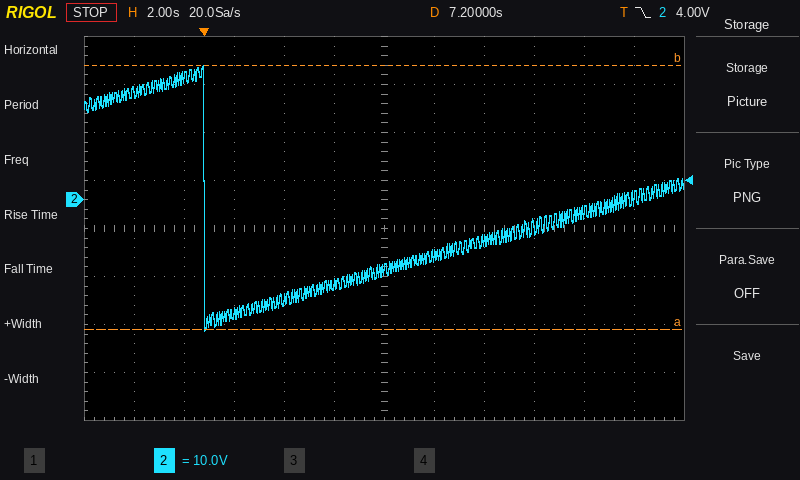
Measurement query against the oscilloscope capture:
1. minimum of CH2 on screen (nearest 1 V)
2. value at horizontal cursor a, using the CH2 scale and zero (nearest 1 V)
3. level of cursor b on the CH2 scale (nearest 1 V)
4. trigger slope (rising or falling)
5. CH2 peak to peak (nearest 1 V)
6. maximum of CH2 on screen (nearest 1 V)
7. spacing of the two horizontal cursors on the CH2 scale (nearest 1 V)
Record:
-27 V
-27 V
28 V
falling
55 V
28 V
55 V
